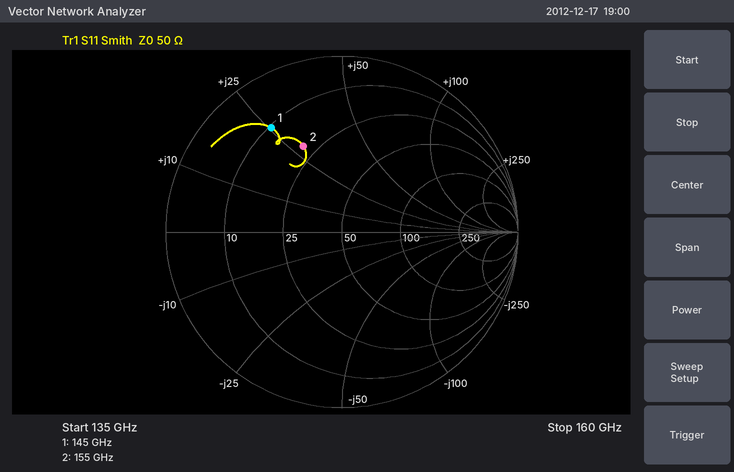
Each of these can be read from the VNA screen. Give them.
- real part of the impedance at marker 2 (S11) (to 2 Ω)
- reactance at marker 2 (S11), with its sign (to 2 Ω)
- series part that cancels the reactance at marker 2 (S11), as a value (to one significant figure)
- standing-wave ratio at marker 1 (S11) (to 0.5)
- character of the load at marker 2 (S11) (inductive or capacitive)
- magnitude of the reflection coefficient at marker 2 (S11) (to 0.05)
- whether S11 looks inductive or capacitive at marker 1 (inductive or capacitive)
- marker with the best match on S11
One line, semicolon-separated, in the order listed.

20 Ω; +28 Ω; 40 fF; 6.0; inductive; 0.55; inductive; marker 2
